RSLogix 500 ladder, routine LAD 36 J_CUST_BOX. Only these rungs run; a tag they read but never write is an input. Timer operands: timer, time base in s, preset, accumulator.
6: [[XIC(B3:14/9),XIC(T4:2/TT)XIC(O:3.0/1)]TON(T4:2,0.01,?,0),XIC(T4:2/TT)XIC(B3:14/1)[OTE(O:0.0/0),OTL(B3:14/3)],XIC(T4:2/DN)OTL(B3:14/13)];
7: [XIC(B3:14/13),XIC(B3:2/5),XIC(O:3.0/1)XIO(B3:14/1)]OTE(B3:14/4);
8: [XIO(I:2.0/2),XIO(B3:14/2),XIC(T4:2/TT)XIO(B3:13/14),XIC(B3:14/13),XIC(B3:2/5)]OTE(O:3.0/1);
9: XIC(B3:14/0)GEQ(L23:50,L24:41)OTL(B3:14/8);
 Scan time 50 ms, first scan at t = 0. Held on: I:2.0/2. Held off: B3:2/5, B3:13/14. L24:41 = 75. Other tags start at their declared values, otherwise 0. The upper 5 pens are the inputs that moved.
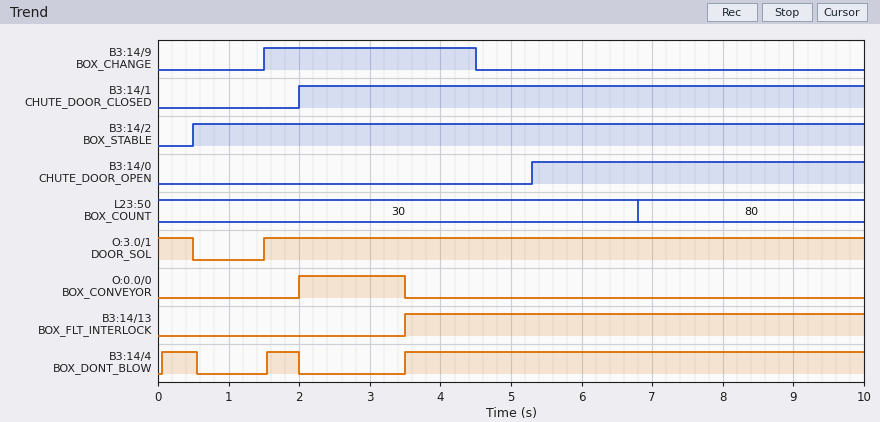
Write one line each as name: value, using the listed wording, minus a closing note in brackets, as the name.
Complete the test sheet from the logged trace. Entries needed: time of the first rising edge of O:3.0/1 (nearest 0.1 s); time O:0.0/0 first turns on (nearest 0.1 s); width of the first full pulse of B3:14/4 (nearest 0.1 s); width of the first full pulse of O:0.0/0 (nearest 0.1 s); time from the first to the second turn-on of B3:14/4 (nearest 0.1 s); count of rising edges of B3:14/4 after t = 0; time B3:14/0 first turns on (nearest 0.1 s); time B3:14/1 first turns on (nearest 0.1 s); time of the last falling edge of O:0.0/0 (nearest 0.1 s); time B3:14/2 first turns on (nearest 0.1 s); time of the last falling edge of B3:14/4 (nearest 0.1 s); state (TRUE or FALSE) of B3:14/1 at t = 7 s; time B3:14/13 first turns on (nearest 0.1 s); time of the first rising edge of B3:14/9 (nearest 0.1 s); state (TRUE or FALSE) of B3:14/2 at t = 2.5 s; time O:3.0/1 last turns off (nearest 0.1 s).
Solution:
time of the first rising edge of O:3.0/1: 1.5 s
time O:0.0/0 first turns on: 2.0 s
width of the first full pulse of B3:14/4: 0.5 s
width of the first full pulse of O:0.0/0: 1.5 s
time from the first to the second turn-on of B3:14/4: 1.5 s
count of rising edges of B3:14/4 after t = 0: 3
time B3:14/0 first turns on: 5.3 s
time B3:14/1 first turns on: 2.0 s
time of the last falling edge of O:0.0/0: 3.5 s
time B3:14/2 first turns on: 0.5 s
time of the last falling edge of B3:14/4: 2.0 s
state (TRUE or FALSE) of B3:14/1 at t = 7 s: TRUE
time B3:14/13 first turns on: 3.5 s
time of the first rising edge of B3:14/9: 1.5 s
state (TRUE or FALSE) of B3:14/2 at t = 2.5 s: TRUE
time O:3.0/1 last turns off: 0.5 s
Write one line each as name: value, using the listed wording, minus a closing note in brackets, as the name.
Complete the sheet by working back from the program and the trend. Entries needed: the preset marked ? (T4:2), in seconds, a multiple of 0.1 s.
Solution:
the preset marked ? (T4:2), in seconds, a multiple of 0.1 s: 2.0 s
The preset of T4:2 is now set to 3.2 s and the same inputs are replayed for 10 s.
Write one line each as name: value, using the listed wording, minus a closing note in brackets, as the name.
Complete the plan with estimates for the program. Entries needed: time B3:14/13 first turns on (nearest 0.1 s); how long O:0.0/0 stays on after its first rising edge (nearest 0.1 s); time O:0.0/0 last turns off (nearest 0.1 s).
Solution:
time B3:14/13 first turns on: 4.7 s
how long O:0.0/0 stays on after its first rising edge: 2.7 s
time O:0.0/0 last turns off: 4.7 s
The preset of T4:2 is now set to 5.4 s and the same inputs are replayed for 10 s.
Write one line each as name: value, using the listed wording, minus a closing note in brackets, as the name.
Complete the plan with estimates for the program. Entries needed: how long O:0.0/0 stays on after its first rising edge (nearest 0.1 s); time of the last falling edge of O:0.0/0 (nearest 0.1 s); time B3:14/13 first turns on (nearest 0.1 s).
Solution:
how long O:0.0/0 stays on after its first rising edge: 4.9 s
time of the last falling edge of O:0.0/0: 6.9 s
time B3:14/13 first turns on: 6.9 s
